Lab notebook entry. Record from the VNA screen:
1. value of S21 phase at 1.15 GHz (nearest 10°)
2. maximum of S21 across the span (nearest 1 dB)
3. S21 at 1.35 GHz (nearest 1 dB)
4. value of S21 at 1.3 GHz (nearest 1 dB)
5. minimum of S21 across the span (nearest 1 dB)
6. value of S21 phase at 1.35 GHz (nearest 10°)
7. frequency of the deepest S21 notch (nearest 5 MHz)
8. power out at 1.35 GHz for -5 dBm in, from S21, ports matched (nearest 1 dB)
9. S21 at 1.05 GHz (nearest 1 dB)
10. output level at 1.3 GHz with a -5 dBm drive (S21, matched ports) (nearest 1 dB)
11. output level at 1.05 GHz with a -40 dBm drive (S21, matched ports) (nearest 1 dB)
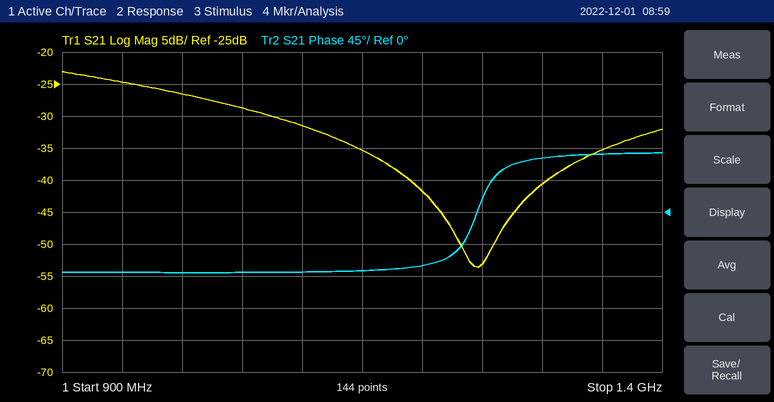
-80°
-23 dB
-35 dB
-41 dB
-54 dB
80°
1.245 GHz
-40 dBm
-29 dB
-46 dBm
-69 dBm
